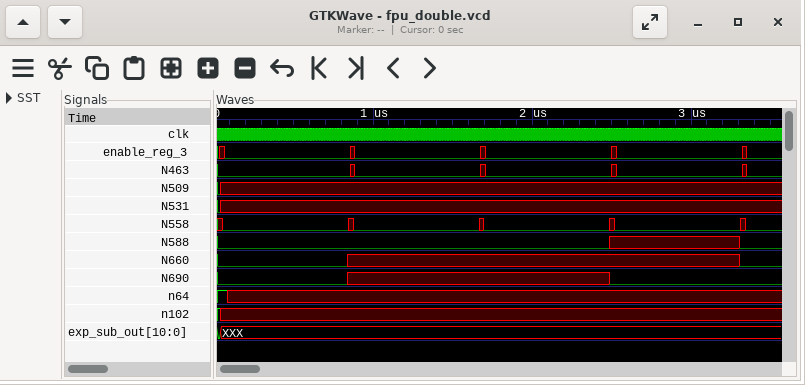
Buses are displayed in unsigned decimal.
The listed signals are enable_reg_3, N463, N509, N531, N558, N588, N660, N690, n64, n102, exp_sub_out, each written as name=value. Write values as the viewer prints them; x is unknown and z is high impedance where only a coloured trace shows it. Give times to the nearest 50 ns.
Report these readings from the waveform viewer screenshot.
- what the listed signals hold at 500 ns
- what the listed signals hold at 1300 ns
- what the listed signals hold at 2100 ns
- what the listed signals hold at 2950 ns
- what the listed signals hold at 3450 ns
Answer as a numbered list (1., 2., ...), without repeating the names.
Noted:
1. enable_reg_3=0, N463=0, N509=x, N531=x, N558=0, N588=0, N660=0, N690=0, n64=x, n102=x, exp_sub_out=XXX
2. enable_reg_3=0, N463=0, N509=x, N531=x, N558=0, N588=0, N660=x, N690=x, n64=x, n102=x, exp_sub_out=XXX
3. enable_reg_3=0, N463=0, N509=x, N531=x, N558=0, N588=0, N660=x, N690=x, n64=x, n102=x, exp_sub_out=XXX
4. enable_reg_3=0, N463=0, N509=x, N531=x, N558=0, N588=x, N660=x, N690=0, n64=x, n102=x, exp_sub_out=XXX
5. enable_reg_3=0, N463=0, N509=x, N531=x, N558=0, N588=0, N660=0, N690=0, n64=x, n102=x, exp_sub_out=XXX
